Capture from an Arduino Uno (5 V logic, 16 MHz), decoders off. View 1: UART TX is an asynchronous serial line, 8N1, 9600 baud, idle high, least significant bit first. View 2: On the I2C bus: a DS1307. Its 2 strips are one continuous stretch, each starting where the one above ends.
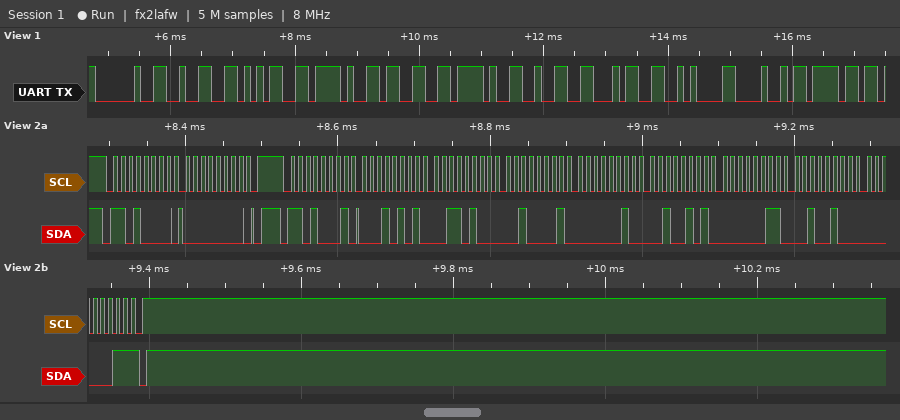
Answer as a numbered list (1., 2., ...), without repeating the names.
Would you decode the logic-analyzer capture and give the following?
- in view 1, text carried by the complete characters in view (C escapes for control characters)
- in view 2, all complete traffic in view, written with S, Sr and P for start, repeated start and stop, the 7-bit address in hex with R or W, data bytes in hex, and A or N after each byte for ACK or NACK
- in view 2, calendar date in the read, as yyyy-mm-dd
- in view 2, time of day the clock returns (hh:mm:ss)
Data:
1. " 25/3/24\nHo"
2. S 68W A 00 A P S 68R A 15 A 34 A 21 A 02 A 25 A 03 A 24 A 03 N P
3. 2024-03-25
4. 21:34:15
